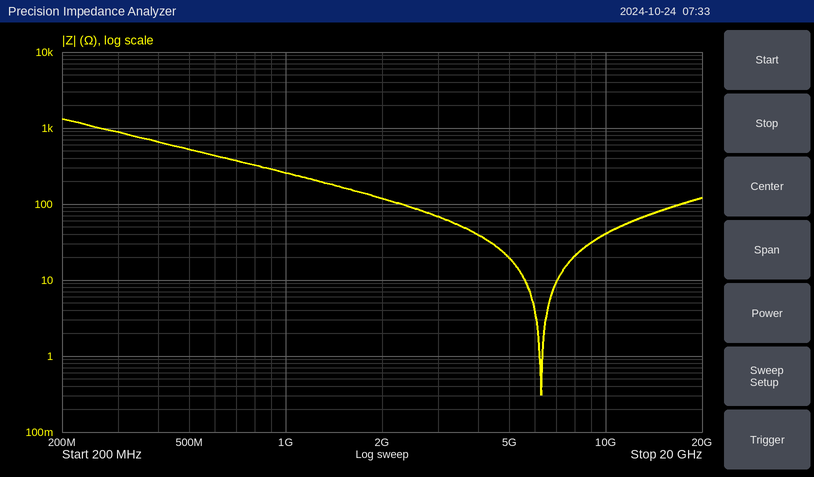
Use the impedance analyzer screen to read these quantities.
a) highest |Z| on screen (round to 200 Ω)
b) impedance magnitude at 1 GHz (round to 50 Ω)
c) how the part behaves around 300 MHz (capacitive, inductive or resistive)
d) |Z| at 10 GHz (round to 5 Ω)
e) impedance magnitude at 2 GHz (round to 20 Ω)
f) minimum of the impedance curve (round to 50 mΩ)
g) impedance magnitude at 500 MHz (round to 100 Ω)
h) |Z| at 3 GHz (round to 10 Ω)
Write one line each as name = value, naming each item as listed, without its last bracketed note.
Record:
highest |Z| on screen = 1.4 kΩ
impedance magnitude at 1 GHz = 250 Ω
how the part behaves around 300 MHz = capacitive
|Z| at 10 GHz = 40 Ω
impedance magnitude at 2 GHz = 120 Ω
minimum of the impedance curve = 300 mΩ
impedance magnitude at 500 MHz = 500 Ω
|Z| at 3 GHz = 70 Ω
